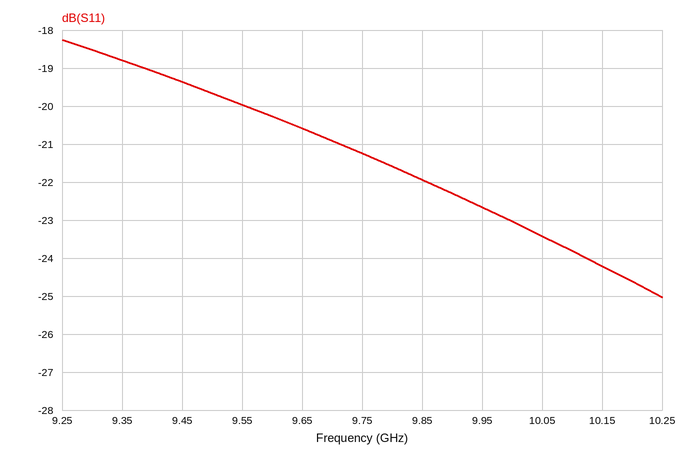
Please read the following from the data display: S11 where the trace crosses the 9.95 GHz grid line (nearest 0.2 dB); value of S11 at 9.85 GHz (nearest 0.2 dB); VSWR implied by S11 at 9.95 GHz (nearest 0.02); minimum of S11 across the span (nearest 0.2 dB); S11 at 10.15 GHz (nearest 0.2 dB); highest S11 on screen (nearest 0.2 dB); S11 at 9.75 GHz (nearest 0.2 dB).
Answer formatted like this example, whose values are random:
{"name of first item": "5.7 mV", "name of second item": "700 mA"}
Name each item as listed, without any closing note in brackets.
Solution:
{"S11 where the trace crosses the 9.95 GHz grid line": "-22.6 dB", "value of S11 at 9.85 GHz": "-22.0 dB", "VSWR implied by S11 at 9.95 GHz": "1.16", "minimum of S11 across the span": "-25.0 dB", "S11 at 10.15 GHz": "-24.2 dB", "highest S11 on screen": "-18.2 dB", "S11 at 9.75 GHz": "-21.2 dB"}
